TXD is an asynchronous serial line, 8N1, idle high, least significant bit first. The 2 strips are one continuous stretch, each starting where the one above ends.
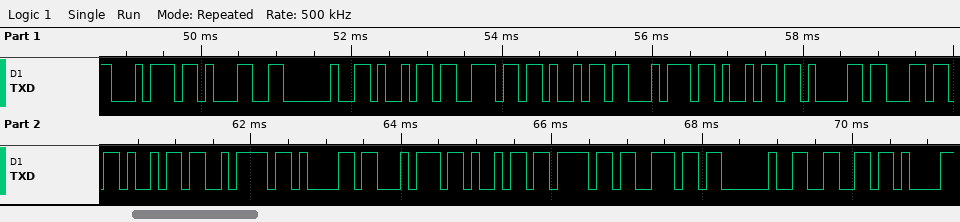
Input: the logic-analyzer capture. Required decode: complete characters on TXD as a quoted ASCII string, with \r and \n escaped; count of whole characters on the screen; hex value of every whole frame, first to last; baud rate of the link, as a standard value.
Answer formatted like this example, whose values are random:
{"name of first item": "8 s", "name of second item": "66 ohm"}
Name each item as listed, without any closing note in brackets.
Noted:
{"complete characters on TXD as a quoted ASCII string, with \\r and \\n escaped": "\"t1 initialization f\"", "count of whole characters on the screen": "19", "hex value of every whole frame, first to last": "74 31 20 69 6E 69 74 69 61 6C 69 7A 61 74 69 6F 6E 20 66", "baud rate of the link, as a standard value": "9600 baud"}
